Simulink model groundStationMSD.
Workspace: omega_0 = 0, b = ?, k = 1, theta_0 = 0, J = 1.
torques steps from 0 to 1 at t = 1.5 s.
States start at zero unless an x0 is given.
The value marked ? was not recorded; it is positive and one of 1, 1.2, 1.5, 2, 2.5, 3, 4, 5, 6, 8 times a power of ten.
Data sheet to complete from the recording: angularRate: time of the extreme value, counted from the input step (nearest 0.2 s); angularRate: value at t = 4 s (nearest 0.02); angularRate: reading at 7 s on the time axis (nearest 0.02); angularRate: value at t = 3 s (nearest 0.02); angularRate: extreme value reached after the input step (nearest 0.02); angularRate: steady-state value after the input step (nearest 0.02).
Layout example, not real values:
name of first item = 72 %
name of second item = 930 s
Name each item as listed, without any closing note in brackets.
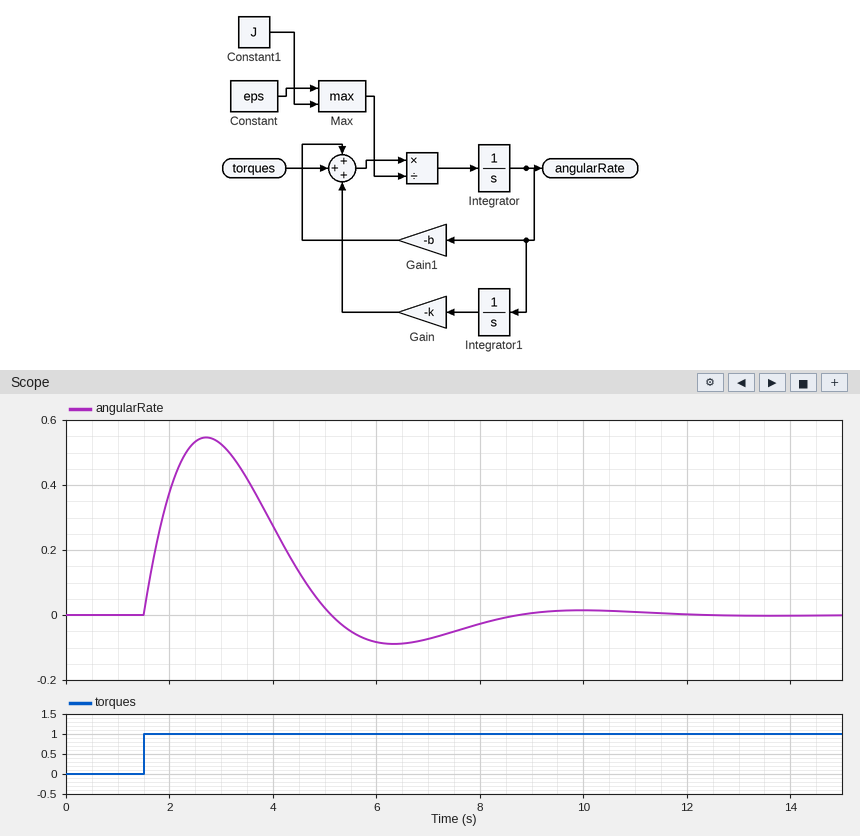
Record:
angularRate: time of the extreme value, counted from the input step = 1.2 s
angularRate: value at t = 4 s = 0.28
angularRate: reading at 7 s on the time axis = -0.08
angularRate: value at t = 3 s = 0.52
angularRate: extreme value reached after the input step = 0.54
angularRate: steady-state value after the input step = 0.00
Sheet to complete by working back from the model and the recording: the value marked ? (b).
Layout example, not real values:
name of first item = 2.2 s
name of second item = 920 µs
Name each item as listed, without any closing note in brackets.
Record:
the value marked ? = 1
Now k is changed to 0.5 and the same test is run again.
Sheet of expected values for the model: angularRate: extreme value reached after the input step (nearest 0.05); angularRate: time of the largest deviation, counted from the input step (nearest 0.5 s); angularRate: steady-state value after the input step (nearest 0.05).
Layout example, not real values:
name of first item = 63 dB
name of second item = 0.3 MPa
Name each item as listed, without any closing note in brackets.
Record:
angularRate: extreme value reached after the input step = 0.65
angularRate: time of the largest deviation, counted from the input step = 1.5 s
angularRate: steady-state value after the input step = 0.00
